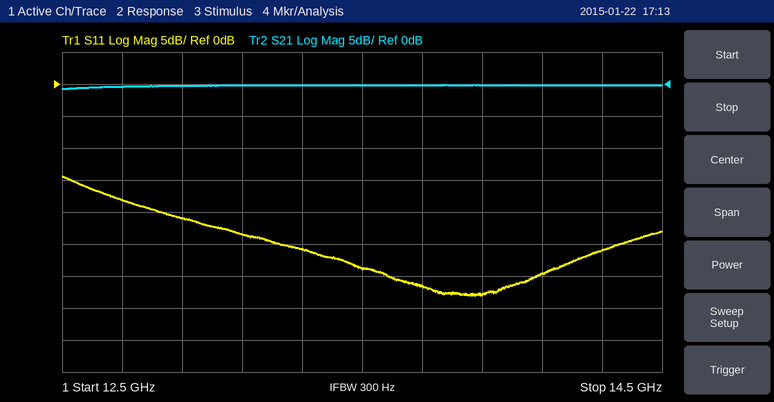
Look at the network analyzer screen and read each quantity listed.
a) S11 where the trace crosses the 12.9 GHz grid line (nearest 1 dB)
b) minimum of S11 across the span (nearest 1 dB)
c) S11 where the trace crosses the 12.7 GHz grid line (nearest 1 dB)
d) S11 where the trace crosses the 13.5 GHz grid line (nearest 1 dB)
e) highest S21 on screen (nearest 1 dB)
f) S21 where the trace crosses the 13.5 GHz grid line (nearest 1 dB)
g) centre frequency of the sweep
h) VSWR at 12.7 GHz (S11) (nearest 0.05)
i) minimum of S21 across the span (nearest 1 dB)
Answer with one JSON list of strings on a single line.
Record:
["-21 dB", "-33 dB", "-18 dB", "-29 dB", "0 dB", "0 dB", "13.5 GHz", "1.30", "-1 dB"]
